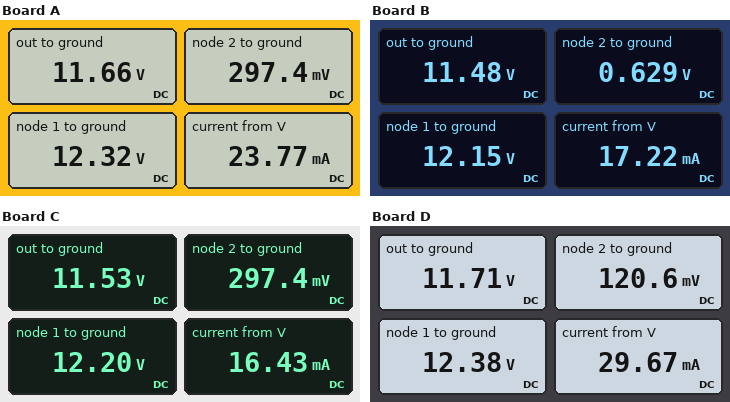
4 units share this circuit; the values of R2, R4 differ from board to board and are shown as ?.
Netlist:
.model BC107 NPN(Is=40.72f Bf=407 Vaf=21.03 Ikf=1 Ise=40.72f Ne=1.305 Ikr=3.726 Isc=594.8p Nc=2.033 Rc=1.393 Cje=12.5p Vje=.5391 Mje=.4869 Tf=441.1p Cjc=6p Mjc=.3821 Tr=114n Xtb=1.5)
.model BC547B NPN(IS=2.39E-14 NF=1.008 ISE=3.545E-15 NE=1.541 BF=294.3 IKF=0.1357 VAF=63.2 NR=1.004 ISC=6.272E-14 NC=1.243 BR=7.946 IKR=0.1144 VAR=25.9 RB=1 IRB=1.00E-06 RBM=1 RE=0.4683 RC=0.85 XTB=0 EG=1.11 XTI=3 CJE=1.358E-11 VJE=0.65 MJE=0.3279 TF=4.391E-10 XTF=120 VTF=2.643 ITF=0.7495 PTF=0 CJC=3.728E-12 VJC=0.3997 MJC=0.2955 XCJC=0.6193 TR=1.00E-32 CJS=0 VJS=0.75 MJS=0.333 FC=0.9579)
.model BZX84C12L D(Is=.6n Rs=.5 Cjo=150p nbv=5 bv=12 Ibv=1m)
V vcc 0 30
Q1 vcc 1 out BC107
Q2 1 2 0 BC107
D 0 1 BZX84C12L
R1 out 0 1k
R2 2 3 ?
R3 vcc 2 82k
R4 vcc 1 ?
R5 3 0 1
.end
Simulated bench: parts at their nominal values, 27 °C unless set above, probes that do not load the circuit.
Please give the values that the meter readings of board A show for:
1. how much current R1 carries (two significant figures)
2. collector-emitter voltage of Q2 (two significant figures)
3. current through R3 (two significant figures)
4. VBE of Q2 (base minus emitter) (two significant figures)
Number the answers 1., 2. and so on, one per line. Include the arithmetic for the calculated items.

1. (11.66 V) / 1 kΩ = 12 mA
2. 12.32 V = 12 V
3. (30 V - 297.4 mV) / 82 kΩ = 360 µA
4. 297.4 mV = 300 mV
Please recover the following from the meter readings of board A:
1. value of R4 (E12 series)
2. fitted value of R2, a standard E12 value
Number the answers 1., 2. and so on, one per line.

1. 1.5 kΩ
2. 820 Ω
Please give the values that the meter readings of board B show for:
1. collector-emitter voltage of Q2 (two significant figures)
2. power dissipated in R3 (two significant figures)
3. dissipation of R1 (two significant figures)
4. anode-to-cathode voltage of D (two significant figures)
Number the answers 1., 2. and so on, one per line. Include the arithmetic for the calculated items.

1. 12.15 V = 12 V
2. (30 V - 629 mV)^2 / 82 kΩ = 11 mW
3. (11.48 V)^2 / 1 kΩ = 130 mW
4. 0 V - 12.15 V = -12 V
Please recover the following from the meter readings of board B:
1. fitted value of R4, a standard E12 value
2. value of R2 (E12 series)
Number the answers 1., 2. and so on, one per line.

1. 3.3 kΩ
2. 1.8 kΩ
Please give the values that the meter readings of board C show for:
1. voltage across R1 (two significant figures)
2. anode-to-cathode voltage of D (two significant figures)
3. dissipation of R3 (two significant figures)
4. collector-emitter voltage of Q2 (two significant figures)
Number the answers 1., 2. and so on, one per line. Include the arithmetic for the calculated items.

1. 11.53 V = 12 V
2. 0 V - 12.2 V = -12 V
3. (30 V - 297.4 mV)^2 / 82 kΩ = 11 mW
4. 12.2 V = 12 V
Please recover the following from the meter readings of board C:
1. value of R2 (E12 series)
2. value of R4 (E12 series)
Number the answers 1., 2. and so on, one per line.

1. 820 Ω
2. 3.9 kΩ
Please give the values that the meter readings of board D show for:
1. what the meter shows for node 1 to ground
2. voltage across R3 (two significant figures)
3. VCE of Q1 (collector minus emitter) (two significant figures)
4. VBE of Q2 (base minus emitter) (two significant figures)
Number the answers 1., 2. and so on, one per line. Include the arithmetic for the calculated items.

1. 12.38 V
2. 30 V - 120.6 mV = 30 V
3. 30 V - 11.71 V = 18 V
4. 120.6 mV = 120 mV
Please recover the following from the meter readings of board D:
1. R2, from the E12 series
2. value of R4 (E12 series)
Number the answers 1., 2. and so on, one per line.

1. 330 Ω
2. 1 kΩ
